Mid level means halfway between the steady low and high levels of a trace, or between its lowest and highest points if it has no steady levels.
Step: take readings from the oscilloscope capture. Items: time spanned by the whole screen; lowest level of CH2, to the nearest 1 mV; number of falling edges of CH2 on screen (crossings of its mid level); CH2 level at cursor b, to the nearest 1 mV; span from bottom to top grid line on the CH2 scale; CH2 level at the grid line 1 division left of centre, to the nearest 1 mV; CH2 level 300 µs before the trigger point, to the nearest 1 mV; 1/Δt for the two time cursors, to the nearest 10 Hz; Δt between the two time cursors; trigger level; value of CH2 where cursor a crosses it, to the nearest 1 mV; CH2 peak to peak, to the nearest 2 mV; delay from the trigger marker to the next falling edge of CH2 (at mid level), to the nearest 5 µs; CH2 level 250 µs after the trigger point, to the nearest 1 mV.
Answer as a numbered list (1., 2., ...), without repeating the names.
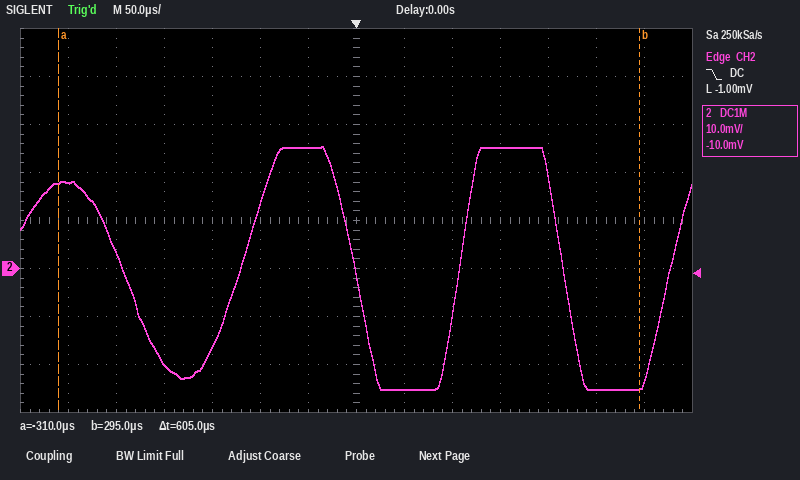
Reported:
1. 700 µs
2. -25 mV
3. 3
4. -25 mV
5. 80 mV
6. 25 mV
7. 18 mV
8. 1.65 kHz
9. 605 µs
10. -1.00 mV
11. 18 mV
12. 50 mV
13. 215 µs
14. -25 mV
